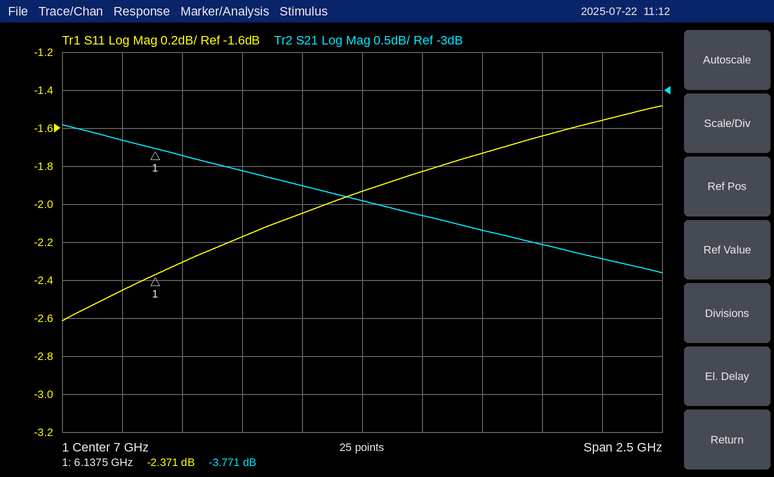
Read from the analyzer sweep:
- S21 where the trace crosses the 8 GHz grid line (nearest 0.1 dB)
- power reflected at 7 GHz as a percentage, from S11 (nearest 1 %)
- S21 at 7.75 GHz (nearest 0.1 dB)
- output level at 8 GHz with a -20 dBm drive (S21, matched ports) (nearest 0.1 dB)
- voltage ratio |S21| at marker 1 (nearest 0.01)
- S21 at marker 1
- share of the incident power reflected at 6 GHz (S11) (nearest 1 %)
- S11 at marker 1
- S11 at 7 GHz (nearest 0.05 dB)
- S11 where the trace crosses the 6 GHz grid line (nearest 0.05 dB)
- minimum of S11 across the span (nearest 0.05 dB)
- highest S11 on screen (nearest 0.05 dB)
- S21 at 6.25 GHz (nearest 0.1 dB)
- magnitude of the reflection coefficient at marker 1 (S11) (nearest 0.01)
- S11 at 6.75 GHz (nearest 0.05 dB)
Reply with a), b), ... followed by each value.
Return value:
a) -5.2 dB
b) 64 %
c) -5.0 dB
d) -25.2 dBm
e) 0.65
f) -3.771 dB
g) 57 %
h) -2.371 dB
i) -1.95 dB
j) -2.45 dB
k) -2.60 dB
l) -1.50 dB
m) -3.9 dB
n) 0.76
o) -2.05 dB
